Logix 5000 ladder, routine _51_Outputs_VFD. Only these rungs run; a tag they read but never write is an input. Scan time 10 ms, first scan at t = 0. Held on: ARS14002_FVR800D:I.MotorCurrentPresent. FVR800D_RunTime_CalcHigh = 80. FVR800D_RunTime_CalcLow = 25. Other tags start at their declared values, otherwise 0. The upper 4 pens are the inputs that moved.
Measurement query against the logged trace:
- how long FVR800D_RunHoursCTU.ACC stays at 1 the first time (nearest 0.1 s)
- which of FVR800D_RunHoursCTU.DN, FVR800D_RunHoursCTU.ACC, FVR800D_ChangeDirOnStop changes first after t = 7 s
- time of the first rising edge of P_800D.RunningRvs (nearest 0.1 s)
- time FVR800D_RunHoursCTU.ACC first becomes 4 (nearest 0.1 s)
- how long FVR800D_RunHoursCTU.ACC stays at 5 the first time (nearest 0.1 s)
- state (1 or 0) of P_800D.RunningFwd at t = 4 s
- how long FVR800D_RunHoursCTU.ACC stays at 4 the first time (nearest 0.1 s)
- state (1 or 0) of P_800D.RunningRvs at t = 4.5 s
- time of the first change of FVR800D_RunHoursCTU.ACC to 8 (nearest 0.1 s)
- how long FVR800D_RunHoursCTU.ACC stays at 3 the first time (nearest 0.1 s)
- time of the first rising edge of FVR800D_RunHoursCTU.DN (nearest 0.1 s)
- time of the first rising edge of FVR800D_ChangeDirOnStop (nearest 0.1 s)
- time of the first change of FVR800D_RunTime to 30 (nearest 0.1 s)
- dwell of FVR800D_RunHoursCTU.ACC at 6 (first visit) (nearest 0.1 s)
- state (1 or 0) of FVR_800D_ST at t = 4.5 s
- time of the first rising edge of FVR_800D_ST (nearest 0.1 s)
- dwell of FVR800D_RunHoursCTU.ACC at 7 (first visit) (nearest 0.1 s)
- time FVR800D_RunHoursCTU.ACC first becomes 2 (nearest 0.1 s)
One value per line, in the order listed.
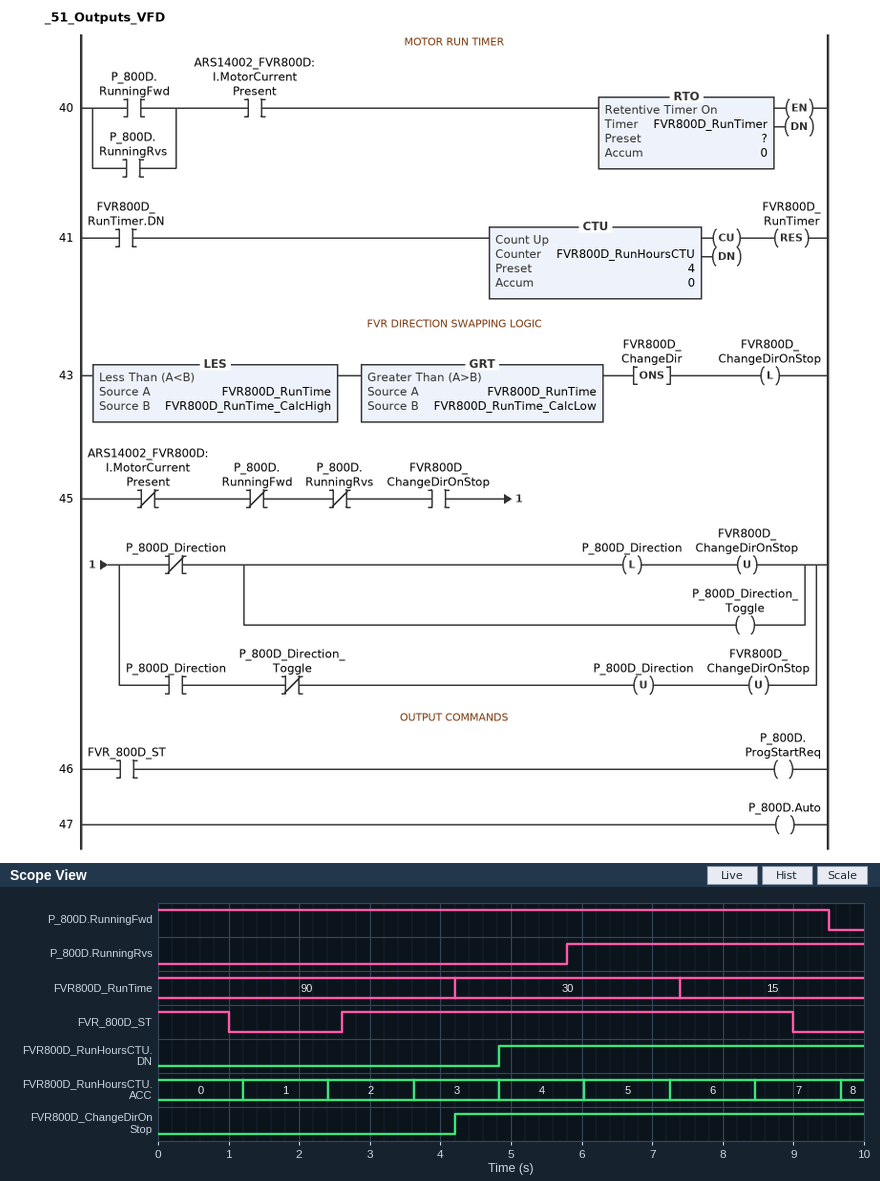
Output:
1.2 s
FVR800D_RunHoursCTU.ACC
5.8 s
4.8 s
1.2 s
1
1.2 s
0
9.7 s
1.2 s
4.8 s
4.2 s
4.2 s
1.2 s
1
2.6 s
1.2 s
2.4 s
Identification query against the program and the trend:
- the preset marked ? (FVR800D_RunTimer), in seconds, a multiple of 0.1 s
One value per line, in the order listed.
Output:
1.2 s
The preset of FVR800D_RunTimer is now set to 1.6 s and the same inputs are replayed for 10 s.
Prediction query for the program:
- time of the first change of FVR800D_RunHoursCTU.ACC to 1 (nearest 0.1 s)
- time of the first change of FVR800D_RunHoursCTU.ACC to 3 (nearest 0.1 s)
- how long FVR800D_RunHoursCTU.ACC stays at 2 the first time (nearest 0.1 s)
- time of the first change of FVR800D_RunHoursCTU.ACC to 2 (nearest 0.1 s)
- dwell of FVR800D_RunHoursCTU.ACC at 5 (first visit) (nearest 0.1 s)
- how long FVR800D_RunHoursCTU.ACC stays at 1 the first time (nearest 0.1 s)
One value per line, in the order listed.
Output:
1.6 s
4.8 s
1.6 s
3.2 s
1.6 s
1.6 s
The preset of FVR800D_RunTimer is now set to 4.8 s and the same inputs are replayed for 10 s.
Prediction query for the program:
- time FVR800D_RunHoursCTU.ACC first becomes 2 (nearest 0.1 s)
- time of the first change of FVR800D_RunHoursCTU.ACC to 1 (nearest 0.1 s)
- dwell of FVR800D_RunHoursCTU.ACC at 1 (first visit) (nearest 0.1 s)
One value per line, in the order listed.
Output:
9.6 s
4.8 s
4.8 s
